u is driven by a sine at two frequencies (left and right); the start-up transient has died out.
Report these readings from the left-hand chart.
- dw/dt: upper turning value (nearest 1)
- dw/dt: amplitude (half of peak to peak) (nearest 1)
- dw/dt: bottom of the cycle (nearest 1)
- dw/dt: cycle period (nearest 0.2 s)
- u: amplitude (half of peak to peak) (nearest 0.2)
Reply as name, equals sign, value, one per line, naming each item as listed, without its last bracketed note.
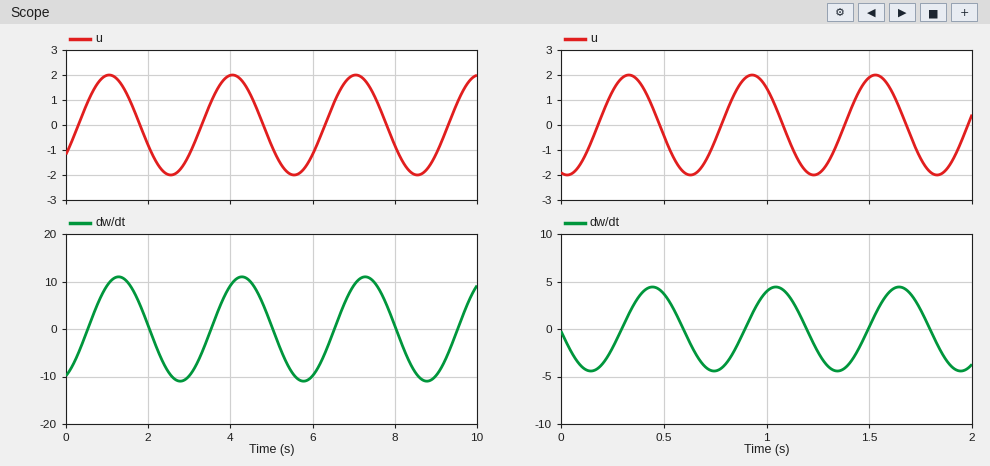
dw/dt: upper turning value = 11
dw/dt: amplitude (half of peak to peak) = 11
dw/dt: bottom of the cycle = -11
dw/dt: cycle period = 3.0 s
u: amplitude (half of peak to peak) = 2.0
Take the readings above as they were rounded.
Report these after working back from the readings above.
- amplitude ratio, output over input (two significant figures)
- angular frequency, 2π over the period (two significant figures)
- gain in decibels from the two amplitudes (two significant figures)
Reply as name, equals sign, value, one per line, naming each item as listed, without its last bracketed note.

amplitude ratio, output over input = 5.5
angular frequency, 2π over the period = 2.1 rad/s
gain in decibels from the two amplitudes = 15 dB
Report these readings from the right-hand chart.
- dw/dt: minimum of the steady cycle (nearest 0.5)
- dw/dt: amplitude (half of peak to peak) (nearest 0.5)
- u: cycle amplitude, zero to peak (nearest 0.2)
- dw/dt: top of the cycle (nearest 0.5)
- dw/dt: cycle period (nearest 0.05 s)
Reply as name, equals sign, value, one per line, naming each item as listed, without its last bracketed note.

dw/dt: minimum of the steady cycle = -4.5
dw/dt: amplitude (half of peak to peak) = 4.5
u: cycle amplitude, zero to peak = 2.0
dw/dt: top of the cycle = 4.5
dw/dt: cycle period = 0.60 s
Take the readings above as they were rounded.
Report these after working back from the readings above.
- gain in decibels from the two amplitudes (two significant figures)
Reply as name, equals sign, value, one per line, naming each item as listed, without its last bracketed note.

gain in decibels from the two amplitudes = 7.0 dB
